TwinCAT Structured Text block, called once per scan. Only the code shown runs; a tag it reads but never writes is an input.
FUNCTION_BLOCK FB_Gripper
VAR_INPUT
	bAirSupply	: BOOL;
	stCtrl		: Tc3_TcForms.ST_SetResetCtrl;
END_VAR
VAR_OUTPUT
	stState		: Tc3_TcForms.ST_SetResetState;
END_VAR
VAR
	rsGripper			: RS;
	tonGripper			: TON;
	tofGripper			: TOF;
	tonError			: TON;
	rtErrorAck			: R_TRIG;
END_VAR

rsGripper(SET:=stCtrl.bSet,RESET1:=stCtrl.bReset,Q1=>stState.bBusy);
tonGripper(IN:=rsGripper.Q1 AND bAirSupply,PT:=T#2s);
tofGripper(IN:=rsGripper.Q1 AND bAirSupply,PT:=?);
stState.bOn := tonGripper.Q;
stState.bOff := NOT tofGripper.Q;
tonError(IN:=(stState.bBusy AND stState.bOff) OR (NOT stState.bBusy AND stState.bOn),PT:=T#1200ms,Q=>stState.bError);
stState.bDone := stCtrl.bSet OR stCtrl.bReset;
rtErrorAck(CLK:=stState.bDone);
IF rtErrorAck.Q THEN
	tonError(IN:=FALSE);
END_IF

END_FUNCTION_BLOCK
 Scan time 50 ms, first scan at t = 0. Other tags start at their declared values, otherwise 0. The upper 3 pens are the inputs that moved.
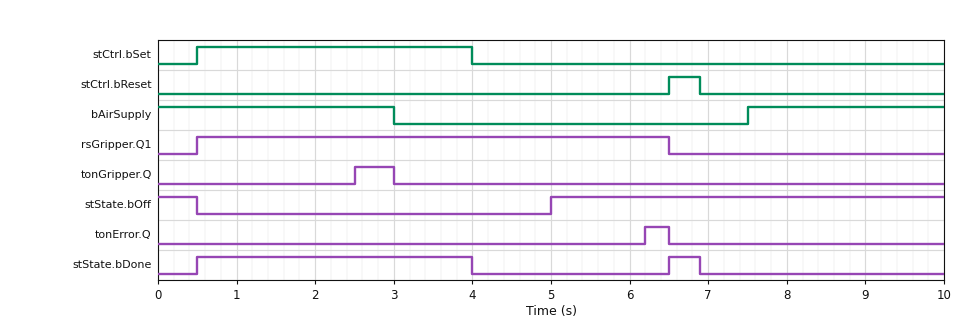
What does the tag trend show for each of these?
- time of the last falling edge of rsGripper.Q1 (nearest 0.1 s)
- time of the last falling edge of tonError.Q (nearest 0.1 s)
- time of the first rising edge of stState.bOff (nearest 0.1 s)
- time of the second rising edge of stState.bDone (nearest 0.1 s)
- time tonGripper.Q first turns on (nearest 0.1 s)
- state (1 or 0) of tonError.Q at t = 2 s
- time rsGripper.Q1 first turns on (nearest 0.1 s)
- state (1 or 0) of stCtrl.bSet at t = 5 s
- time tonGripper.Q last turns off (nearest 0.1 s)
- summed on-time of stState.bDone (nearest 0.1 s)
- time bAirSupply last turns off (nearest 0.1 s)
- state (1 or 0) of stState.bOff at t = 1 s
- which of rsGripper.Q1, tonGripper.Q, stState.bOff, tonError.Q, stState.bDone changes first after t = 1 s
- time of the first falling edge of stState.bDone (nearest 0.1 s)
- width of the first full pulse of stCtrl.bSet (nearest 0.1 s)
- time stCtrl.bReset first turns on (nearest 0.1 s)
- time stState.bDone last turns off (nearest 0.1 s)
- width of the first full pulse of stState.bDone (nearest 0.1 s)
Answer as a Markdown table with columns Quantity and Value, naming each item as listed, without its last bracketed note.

| Quantity | Value |
|---|---|
| time of the last falling edge of rsGripper.Q1 | 6.5 s |
| time of the last falling edge of tonError.Q | 6.5 s |
| time of the first rising edge of stState.bOff | 5.0 s |
| time of the second rising edge of stState.bDone | 6.5 s |
| time tonGripper.Q first turns on | 2.5 s |
| state (1 or 0) of tonError.Q at t = 2 s | 0 |
| time rsGripper.Q1 first turns on | 0.5 s |
| state (1 or 0) of stCtrl.bSet at t = 5 s | 0 |
| time tonGripper.Q last turns off | 3.0 s |
| summed on-time of stState.bDone | 3.9 s |
| time bAirSupply last turns off | 3.0 s |
| state (1 or 0) of stState.bOff at t = 1 s | 0 |
| which of rsGripper.Q1, tonGripper.Q, stState.bOff, tonError.Q, stState.bDone changes first after t = 1 s | tonGripper.Q |
| time of the first falling edge of stState.bDone | 4.0 s |
| width of the first full pulse of stCtrl.bSet | 3.5 s |
| time stCtrl.bReset first turns on | 6.5 s |
| time stState.bDone last turns off | 6.9 s |
| width of the first full pulse of stState.bDone | 3.5 s |
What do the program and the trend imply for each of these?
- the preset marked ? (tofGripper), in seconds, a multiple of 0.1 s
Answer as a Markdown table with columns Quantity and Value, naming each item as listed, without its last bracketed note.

| Quantity | Value |
|---|---|
| the preset marked ? (tofGripper), in seconds, a multiple of 0.1 s | 2.0 s |
